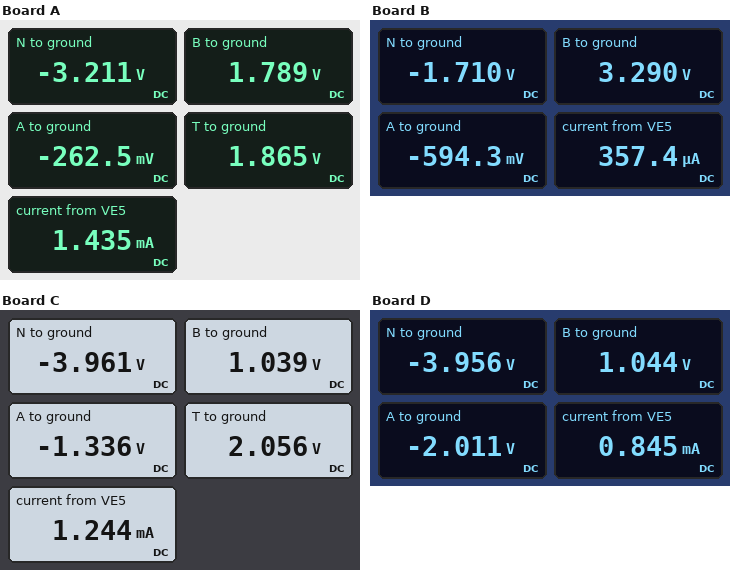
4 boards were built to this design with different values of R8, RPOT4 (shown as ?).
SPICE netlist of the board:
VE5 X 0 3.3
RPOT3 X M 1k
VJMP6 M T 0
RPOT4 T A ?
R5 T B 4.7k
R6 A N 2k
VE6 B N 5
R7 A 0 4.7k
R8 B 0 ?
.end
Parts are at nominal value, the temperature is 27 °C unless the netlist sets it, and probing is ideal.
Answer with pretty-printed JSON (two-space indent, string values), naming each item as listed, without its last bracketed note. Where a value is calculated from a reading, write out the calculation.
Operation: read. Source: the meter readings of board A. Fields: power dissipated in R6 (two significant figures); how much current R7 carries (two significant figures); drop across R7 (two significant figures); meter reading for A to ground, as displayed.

{
  "power dissipated in R6": "(-262.5 mV - (-3.211 V))^2 / 2 kΩ = 4.3 mW",
  "how much current R7 carries": "(0 V - (-262.5 mV)) / 4.7 kΩ = 56 µA",
  "drop across R7": "0 V - (-262.5 mV) = 260 mV",
  "meter reading for A to ground, as displayed": "-262.5 mV"
}
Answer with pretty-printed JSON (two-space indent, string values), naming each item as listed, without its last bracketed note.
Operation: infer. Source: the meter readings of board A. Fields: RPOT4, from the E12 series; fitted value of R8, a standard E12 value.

{
  "RPOT4, from the E12 series": "1.5 kΩ",
  "fitted value of R8, a standard E12 value": "1.2 kΩ"
}
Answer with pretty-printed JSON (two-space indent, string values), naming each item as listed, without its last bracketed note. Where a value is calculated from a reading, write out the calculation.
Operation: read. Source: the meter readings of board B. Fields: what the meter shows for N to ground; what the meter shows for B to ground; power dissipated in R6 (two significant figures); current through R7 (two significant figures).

{
  "what the meter shows for N to ground": "-1.710 V",
  "what the meter shows for B to ground": "3.290 V",
  "power dissipated in R6": "(-594.3 mV - (-1.71 V))^2 / 2 kΩ = 620 µW",
  "current through R7": "(0 V - (-594.3 mV)) / 4.7 kΩ = 130 µA"
}
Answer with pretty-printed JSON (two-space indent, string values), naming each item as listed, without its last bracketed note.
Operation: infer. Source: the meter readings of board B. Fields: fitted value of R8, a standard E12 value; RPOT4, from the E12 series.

{
  "fitted value of R8, a standard E12 value": "6.8 kΩ",
  "RPOT4, from the E12 series": "8.2 kΩ"
}
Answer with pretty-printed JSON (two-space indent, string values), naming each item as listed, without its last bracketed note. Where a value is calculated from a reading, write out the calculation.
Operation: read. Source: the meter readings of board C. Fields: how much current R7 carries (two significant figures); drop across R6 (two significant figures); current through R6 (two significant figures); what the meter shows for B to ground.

{
  "how much current R7 carries": "(0 V - (-1.336 V)) / 4.7 kΩ = 280 µA",
  "drop across R6": "-1.336 V - (-3.961 V) = 2.6 V",
  "current through R6": "(-1.336 V - (-3.961 V)) / 2 kΩ = 1.3 mA",
  "what the meter shows for B to ground": "1.039 V"
}
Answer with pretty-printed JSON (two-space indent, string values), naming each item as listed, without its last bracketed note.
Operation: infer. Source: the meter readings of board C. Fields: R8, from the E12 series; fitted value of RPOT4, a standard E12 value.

{
  "R8, from the E12 series": "680 Ω",
  "fitted value of RPOT4, a standard E12 value": "3.3 kΩ"
}
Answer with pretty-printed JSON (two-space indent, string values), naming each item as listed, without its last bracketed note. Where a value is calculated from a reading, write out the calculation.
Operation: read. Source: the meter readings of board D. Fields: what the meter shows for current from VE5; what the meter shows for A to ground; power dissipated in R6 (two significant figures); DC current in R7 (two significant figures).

{
  "what the meter shows for current from VE5": "0.845 mA",
  "what the meter shows for A to ground": "-2.011 V",
  "power dissipated in R6": "(-2.011 V - (-3.956 V))^2 / 2 kΩ = 1.9 mW",
  "DC current in R7": "(0 V - (-2.011 V)) / 4.7 kΩ = 430 µA"
}
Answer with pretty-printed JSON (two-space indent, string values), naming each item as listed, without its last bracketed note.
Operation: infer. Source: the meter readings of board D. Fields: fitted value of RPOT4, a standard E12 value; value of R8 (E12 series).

{
  "fitted value of RPOT4, a standard E12 value": "8.2 kΩ",
  "value of R8": "820 Ω"
}
